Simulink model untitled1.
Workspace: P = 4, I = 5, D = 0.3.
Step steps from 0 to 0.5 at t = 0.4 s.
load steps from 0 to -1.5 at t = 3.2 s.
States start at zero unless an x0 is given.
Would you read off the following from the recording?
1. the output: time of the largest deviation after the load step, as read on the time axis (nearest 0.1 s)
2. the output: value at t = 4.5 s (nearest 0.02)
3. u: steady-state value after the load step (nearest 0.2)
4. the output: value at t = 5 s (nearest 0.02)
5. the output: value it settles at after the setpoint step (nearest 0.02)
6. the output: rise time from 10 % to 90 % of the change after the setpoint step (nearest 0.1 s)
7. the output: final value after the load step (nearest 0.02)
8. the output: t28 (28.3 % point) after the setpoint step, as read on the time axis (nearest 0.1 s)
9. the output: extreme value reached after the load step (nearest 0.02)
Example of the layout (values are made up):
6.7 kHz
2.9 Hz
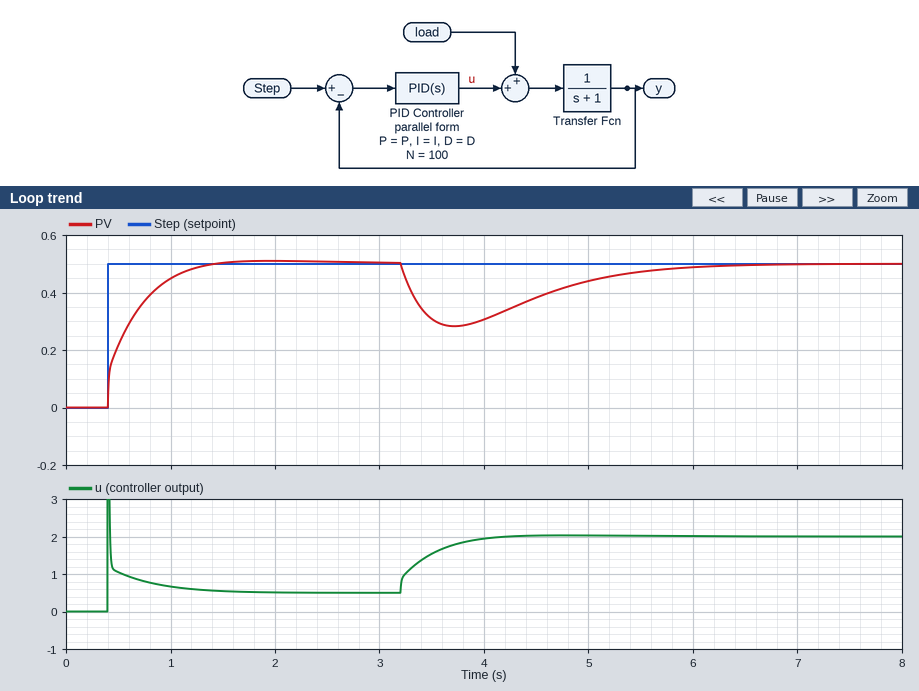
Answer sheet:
3.7 s
0.38
2.0
0.44
0.50
0.6 s
0.50
0.4 s
0.28
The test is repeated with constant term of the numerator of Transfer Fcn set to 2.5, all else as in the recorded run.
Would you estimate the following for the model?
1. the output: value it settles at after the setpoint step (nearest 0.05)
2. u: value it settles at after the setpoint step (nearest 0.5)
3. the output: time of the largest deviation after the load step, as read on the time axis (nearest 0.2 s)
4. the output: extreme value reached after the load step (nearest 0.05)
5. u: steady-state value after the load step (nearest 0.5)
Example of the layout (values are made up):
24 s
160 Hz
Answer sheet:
0.50
0.0
3.6 s
0.25
1.5
